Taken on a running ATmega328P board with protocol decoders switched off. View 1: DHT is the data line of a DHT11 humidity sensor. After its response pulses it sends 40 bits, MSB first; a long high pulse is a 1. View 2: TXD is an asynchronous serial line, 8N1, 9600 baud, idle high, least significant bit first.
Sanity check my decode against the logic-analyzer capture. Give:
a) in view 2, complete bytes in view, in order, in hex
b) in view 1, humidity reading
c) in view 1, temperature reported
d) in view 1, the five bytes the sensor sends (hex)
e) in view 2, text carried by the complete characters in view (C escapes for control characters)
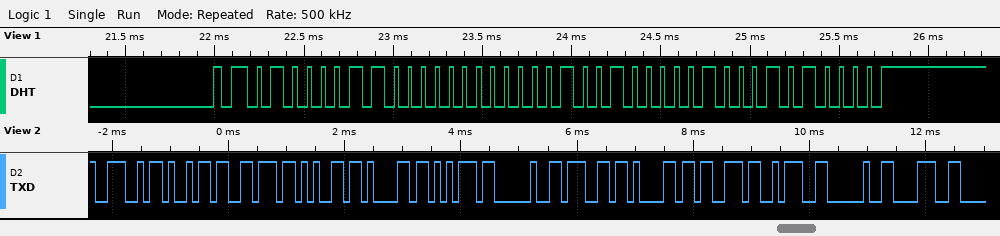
0x4E 0x69 0x76 0x65 0x61 0x75 0x20 0x67 0x61 0x73 0x3A 0x20 0x38
67 %
9.4 °C
43 00 09 04 50
"Niveau gas: 8"
